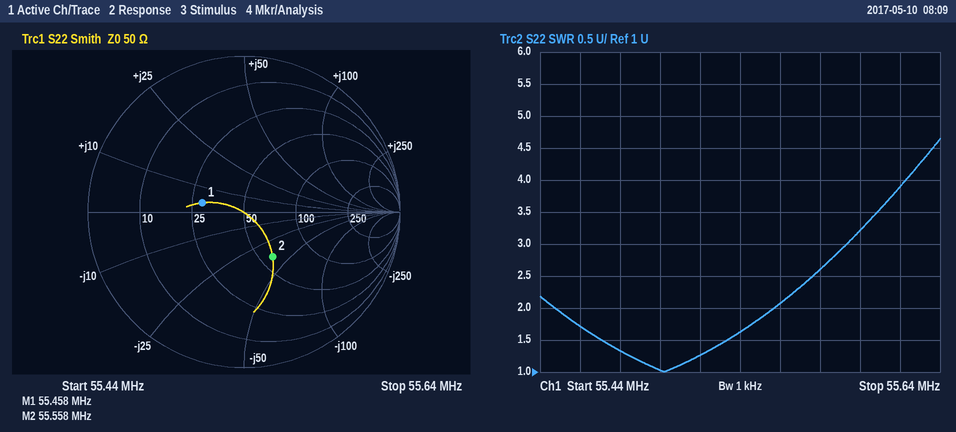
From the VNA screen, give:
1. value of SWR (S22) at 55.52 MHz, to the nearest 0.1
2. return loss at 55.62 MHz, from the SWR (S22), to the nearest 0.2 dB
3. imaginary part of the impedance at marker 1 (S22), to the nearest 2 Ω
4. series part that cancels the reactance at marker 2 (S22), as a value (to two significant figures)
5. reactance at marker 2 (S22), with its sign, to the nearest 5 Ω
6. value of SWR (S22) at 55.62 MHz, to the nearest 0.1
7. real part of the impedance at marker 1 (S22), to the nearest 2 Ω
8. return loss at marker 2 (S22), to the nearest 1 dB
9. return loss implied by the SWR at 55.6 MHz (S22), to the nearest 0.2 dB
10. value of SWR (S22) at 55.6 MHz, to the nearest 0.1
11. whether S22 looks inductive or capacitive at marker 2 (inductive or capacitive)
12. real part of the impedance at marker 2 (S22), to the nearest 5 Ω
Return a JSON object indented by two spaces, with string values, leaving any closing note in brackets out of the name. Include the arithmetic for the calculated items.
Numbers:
{
  "value of SWR (S22) at 55.52 MHz, to the nearest 0.1": "1.3",
  "return loss at 55.62 MHz, from the SWR (S22), to the nearest 0.2 dB": "−20 log10((3.9 − 1)/(3.9 + 1)) ≈ 4.6 dB",
  "imaginary part of the impedance at marker 1 (S22), to the nearest 2 Ω": "+4 Ω",
  "series part that cancels the reactance at marker 2 (S22), as a value": "L = 40 Ω/(2π × 55.558 MHz) ≈ 115 nH, so 110 nH to two significant figures",
  "reactance at marker 2 (S22), with its sign, to the nearest 5 Ω": "-40 Ω",
  "value of SWR (S22) at 55.62 MHz, to the nearest 0.1": "3.9",
  "real part of the impedance at marker 1 (S22), to the nearest 2 Ω": "28 Ω",
  "return loss at marker 2 (S22), to the nearest 1 dB": "9 dB",
  "return loss implied by the SWR at 55.6 MHz (S22), to the nearest 0.2 dB": "−20 log10((3.2 − 1)/(3.2 + 1)) ≈ 5.6 dB",
  "value of SWR (S22) at 55.6 MHz, to the nearest 0.1": "3.2",
  "whether S22 looks inductive or capacitive at marker 2": "capacitive",
  "real part of the impedance at marker 2 (S22), to the nearest 5 Ω": "60 Ω"
}
